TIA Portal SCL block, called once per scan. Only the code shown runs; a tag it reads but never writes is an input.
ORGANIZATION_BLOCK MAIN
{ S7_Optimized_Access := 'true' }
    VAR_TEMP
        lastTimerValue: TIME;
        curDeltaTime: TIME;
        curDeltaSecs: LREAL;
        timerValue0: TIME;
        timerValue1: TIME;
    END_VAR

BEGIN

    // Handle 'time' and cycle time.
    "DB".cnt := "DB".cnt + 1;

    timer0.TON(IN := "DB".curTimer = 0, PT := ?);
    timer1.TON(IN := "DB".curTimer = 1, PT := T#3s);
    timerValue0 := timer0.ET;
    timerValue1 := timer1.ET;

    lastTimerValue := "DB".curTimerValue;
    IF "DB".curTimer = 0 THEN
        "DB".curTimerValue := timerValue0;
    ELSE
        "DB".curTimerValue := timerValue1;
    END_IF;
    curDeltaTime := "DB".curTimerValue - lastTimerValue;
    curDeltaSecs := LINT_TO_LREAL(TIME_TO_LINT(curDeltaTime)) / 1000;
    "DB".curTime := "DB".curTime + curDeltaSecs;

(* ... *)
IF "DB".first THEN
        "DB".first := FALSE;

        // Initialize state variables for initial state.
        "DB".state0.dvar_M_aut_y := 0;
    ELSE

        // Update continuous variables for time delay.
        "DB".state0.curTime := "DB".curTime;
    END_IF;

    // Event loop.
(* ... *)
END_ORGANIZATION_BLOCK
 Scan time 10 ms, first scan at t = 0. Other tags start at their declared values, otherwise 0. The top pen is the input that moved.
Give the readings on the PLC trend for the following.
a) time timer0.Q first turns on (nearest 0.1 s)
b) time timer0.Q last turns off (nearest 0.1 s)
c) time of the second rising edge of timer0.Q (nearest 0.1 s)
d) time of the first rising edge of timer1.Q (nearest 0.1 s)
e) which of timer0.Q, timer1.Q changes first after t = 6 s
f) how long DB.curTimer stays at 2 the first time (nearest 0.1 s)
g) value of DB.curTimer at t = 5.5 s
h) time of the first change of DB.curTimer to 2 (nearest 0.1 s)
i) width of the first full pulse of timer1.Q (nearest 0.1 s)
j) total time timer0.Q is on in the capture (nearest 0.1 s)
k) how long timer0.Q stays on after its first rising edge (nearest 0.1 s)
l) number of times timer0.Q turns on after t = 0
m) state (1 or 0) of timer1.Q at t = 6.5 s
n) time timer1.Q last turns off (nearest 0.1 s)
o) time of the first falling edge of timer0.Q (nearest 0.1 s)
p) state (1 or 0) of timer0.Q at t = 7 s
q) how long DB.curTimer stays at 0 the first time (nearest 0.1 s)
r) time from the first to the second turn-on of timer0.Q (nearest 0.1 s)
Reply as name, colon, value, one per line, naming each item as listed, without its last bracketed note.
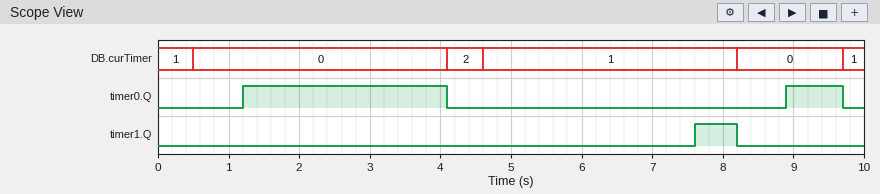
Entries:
time timer0.Q first turns on: 1.2 s
time timer0.Q last turns off: 9.7 s
time of the second rising edge of timer0.Q: 8.9 s
time of the first rising edge of timer1.Q: 7.6 s
which of timer0.Q, timer1.Q changes first after t = 6 s: timer1.Q
how long DB.curTimer stays at 2 the first time: 0.5 s
value of DB.curTimer at t = 5.5 s: 1
time of the first change of DB.curTimer to 2: 4.1 s
width of the first full pulse of timer1.Q: 0.6 s
total time timer0.Q is on in the capture: 3.7 s
how long timer0.Q stays on after its first rising edge: 2.9 s
number of times timer0.Q turns on after t = 0: 2
state (1 or 0) of timer1.Q at t = 6.5 s: 0
time timer1.Q last turns off: 8.2 s
time of the first falling edge of timer0.Q: 4.1 s
state (1 or 0) of timer0.Q at t = 7 s: 0
how long DB.curTimer stays at 0 the first time: 3.6 s
time from the first to the second turn-on of timer0.Q: 7.7 s
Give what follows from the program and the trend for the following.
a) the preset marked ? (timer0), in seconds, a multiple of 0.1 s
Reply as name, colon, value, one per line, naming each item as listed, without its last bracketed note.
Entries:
the preset marked ? (timer0), in seconds, a multiple of 0.1 s: 0.7 s
